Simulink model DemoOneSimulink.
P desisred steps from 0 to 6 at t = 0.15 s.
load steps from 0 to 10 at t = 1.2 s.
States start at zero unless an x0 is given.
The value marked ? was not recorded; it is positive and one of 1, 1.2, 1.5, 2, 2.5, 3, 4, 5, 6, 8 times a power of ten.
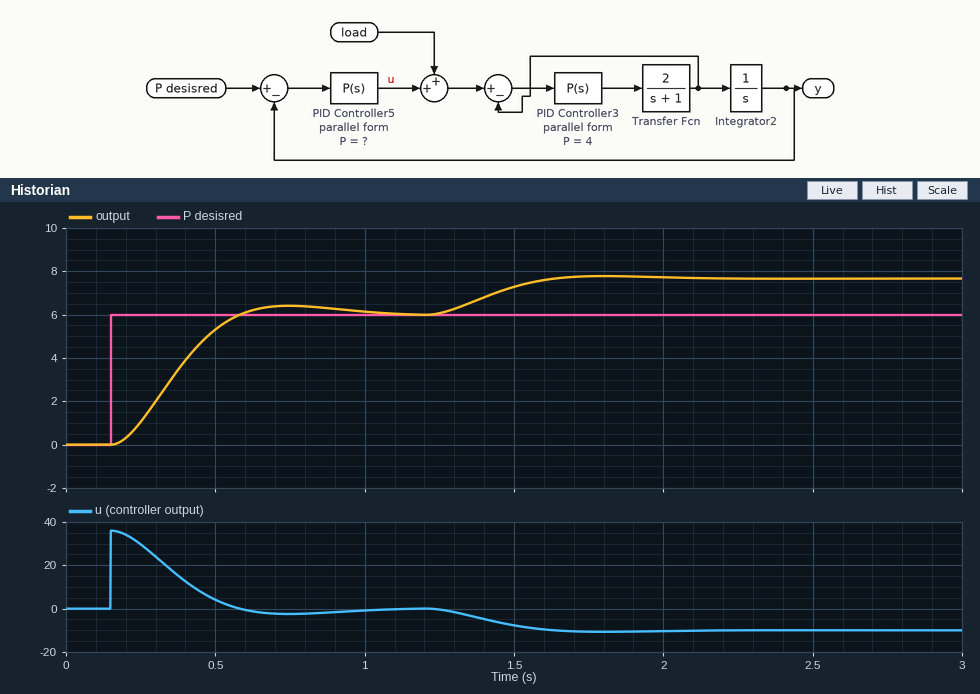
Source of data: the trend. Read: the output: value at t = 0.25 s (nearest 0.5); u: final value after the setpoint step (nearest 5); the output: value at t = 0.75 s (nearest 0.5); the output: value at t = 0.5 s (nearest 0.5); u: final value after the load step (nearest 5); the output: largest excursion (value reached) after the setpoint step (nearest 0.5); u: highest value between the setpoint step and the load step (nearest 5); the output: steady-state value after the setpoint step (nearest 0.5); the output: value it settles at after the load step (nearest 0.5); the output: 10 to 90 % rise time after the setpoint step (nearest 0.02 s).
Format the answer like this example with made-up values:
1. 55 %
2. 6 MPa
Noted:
1. 1.0
2. 0
3. 6.5
4. 5.5
5. -10
6. 6.5
7. 35
8. 6.0
9. 7.5
10. 0.28 s
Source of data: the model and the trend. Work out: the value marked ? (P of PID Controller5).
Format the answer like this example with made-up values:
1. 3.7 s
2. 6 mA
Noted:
1. 6
